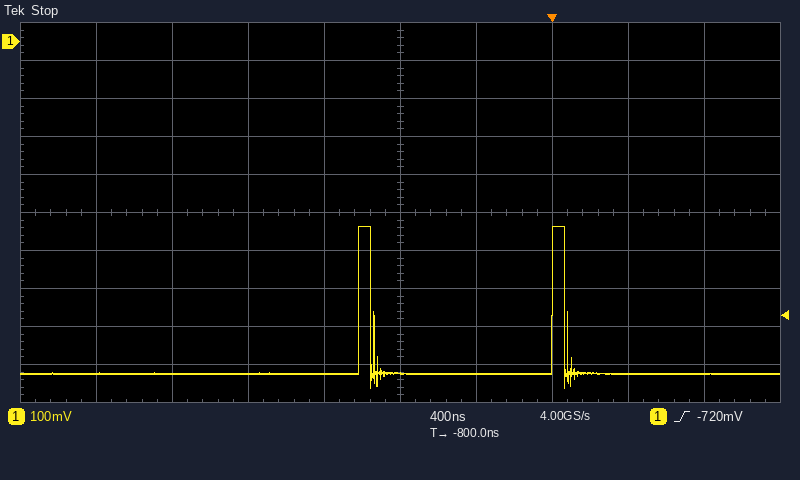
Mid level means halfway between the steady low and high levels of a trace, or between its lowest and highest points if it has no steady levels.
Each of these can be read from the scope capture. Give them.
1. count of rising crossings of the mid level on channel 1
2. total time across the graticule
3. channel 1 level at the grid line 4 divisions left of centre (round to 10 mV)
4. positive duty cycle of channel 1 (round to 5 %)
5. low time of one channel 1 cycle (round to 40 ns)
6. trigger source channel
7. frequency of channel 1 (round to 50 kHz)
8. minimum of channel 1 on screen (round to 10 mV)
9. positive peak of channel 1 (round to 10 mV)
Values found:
2
4 µs
-870 mV
5 %
960 ns
channel 1
1.00 MHz
-910 mV
-490 mV
